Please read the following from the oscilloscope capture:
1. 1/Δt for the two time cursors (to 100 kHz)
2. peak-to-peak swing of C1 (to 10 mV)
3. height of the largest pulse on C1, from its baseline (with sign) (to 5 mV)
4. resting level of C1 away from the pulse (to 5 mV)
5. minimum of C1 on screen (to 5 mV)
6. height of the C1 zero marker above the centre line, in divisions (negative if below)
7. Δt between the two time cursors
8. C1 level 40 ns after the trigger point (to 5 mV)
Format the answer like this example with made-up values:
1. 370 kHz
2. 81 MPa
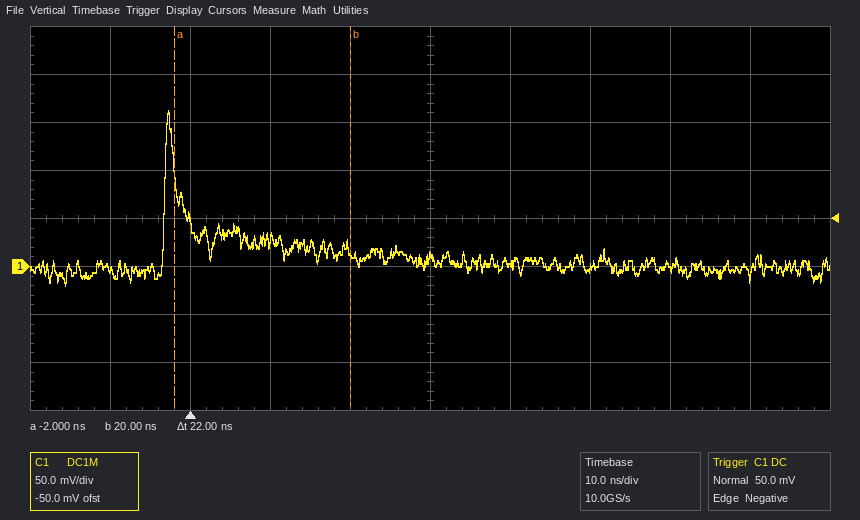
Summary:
1. 45.5 MHz
2. 180 mV
3. +160 mV
4. 0 mV
5. -20 mV
6. -1.0 div
7. 22 ns
8. 0 mV
